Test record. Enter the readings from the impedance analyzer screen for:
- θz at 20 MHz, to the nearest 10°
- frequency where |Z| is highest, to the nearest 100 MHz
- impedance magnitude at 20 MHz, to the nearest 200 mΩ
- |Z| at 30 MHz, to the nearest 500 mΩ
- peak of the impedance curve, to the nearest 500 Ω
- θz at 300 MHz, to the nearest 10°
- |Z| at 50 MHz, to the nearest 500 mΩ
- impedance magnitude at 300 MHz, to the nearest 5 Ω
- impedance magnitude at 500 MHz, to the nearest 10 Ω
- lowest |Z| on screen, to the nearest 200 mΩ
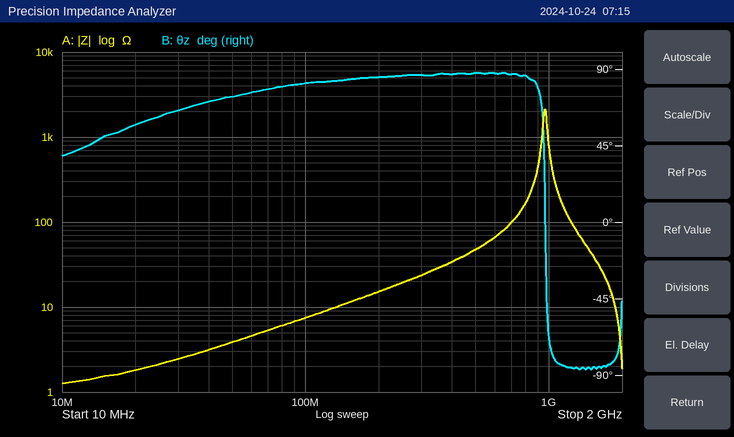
60°
1.0 GHz
1.8 Ω
2.5 Ω
2.0 kΩ
90°
4.0 Ω
25 Ω
50 Ω
1.2 Ω
